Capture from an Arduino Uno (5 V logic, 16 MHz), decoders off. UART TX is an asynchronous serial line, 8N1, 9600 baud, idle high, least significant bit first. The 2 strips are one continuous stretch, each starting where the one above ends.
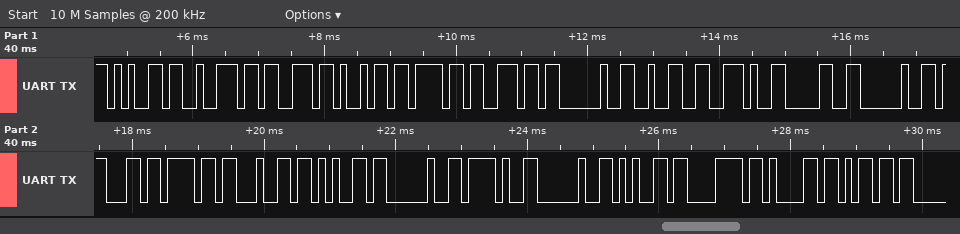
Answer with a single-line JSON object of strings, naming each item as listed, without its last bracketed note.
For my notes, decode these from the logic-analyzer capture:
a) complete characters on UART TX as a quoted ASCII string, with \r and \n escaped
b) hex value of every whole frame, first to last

{"complete characters on UART TX as a quoted ASCII string, with \\r and \\n escaped": "\"ersion 2.0 code / exam\"", "hex value of every whole frame, first to last": "65 72 73 69 6F 6E 20 32 2E 30 20 63 6F 64 65 20 2F 20 65 78 61 6D"}
